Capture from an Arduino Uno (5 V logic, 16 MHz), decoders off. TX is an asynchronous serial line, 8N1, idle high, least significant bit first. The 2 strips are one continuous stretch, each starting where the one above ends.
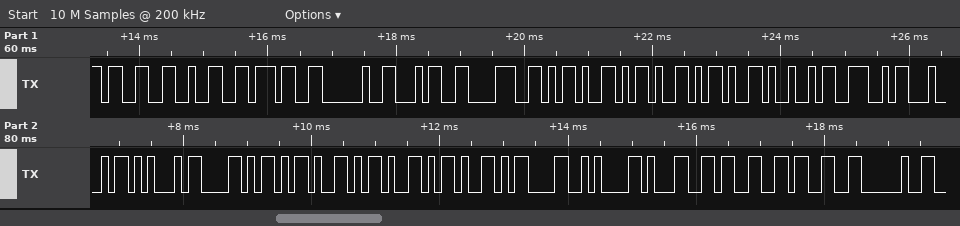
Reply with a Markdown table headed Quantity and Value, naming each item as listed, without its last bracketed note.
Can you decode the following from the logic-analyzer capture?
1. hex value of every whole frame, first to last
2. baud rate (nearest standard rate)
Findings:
| Quantity | Value |
|---|---|
| hex value of every whole frame, first to last | 33 32 37 20 34 38 2D 2D 2D 49 4E 44 45 58 2D 2D 2D 0D 0A 31 33 33 20 |
| baud rate | 9600 baud |
